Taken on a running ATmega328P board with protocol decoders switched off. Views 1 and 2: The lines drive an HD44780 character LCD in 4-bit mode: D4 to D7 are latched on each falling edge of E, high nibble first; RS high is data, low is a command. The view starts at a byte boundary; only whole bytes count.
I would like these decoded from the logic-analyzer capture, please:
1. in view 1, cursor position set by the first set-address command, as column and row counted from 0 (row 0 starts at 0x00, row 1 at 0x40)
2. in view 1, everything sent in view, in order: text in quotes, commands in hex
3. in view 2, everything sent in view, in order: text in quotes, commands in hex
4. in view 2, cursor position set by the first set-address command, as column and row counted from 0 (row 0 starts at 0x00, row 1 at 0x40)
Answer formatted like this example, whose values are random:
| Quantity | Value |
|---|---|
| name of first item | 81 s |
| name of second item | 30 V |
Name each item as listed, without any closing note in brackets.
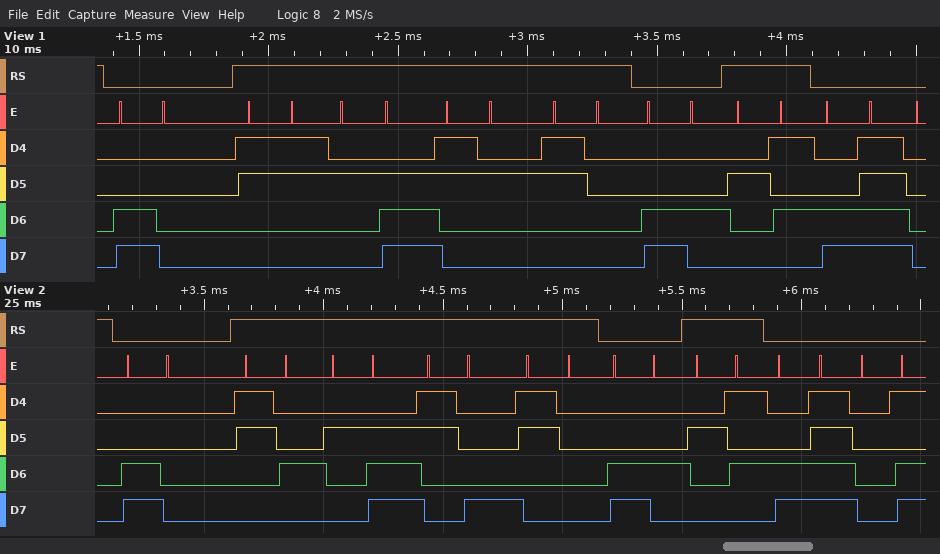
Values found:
| Quantity | Value |
|---|---|
| in view 1, cursor position set by the first set-address command, as column and row counted from 0 | column 0, row 1 |
| in view 1, everything sent in view, in order: text in quotes, commands in hex | 0xC0 "3.20" 0xC4 "%" 0xCF |
| in view 2, everything sent in view, in order: text in quotes, commands in hex | 0xC0 "4.80" 0xC4 "%" 0xCF 0x0D |
| in view 2, cursor position set by the first set-address command, as column and row counted from 0 | column 0, row 1 |
